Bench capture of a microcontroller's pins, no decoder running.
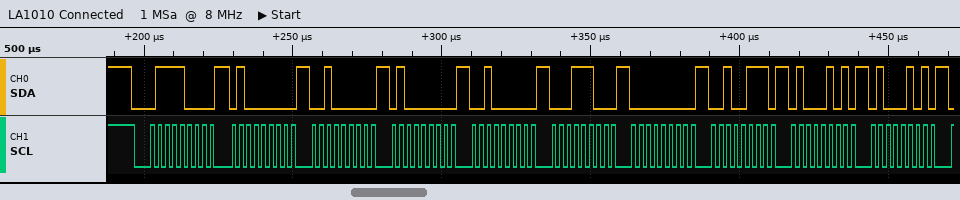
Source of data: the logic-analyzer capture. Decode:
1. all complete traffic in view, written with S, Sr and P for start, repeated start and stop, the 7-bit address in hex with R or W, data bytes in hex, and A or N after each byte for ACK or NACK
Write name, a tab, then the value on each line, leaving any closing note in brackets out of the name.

all complete traffic in view, written with S, Sr and P for start, repeated start and stop, the 7-bit address in hex with R or W, data bytes in hex, and A or N after each byte for ACK or NACK	S 3CW A 40 A 20 A 40 A 20 A 1C A 00 A 27 A 45 A 45 A
